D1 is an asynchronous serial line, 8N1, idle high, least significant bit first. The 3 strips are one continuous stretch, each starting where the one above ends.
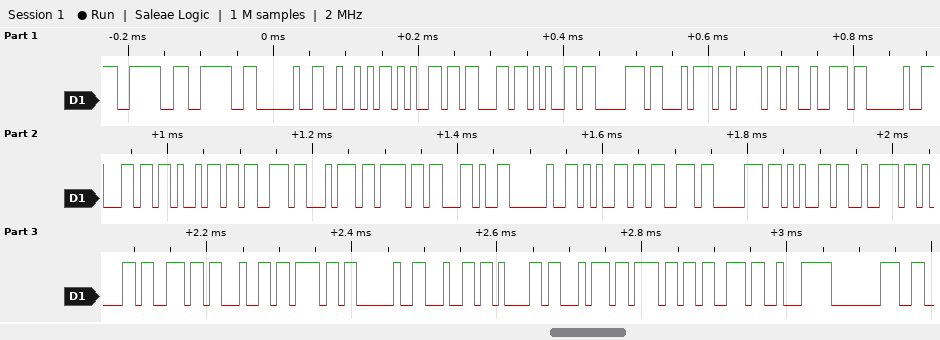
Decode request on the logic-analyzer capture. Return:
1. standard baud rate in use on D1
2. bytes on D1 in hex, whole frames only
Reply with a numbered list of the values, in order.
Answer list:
1. 115200 baud
2. 3E 3E 20 52 65 63 65 70 74 6F 72 20 6C 69 73 74 6F 2C 20 65 73 70 65 72 61 6E 64 6F 20 64 61 74 6F 73 E2 80
